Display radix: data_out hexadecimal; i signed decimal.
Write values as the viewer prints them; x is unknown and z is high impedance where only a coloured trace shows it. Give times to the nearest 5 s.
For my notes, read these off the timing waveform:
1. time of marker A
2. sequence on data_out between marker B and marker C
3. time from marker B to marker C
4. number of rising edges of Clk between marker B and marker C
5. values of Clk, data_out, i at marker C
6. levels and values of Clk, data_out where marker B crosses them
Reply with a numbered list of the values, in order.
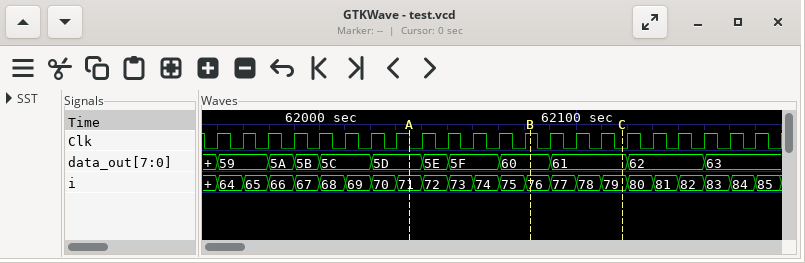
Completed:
1. 62035 s
2. 60, 61
3. 35 s
4. 3
5. Clk=0, data_out=61, i=79
6. Clk=1, data_out=60
